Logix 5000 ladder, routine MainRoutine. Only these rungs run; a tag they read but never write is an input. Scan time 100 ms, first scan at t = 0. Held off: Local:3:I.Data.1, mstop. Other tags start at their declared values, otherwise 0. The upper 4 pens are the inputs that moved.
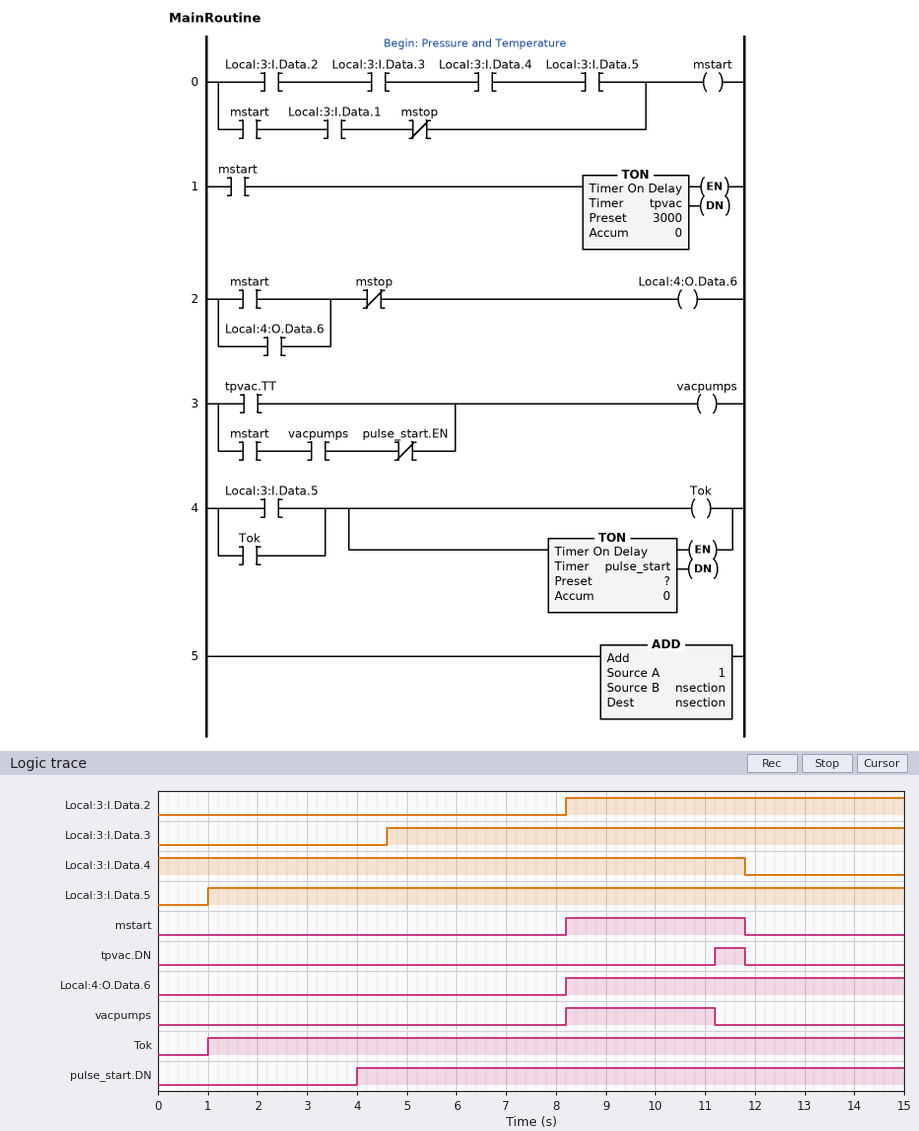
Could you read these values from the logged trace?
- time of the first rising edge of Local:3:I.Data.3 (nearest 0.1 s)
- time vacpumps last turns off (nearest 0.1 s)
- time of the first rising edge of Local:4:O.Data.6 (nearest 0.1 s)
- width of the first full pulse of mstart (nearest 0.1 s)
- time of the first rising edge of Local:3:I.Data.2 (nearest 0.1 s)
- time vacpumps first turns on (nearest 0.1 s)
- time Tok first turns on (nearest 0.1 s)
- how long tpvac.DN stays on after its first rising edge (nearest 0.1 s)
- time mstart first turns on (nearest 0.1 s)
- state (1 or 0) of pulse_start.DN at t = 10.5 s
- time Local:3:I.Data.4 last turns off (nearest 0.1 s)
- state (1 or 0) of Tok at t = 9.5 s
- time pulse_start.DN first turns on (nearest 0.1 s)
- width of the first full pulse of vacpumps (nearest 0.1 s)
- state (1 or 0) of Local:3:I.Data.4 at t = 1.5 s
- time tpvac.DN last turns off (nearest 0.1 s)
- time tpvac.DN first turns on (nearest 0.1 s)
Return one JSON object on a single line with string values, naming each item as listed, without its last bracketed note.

{"time of the first rising edge of Local:3:I.Data.3": "4.6 s", "time vacpumps last turns off": "11.2 s", "time of the first rising edge of Local:4:O.Data.6": "8.2 s", "width of the first full pulse of mstart": "3.6 s", "time of the first rising edge of Local:3:I.Data.2": "8.2 s", "time vacpumps first turns on": "8.2 s", "time Tok first turns on": "1.0 s", "how long tpvac.DN stays on after its first rising edge": "0.6 s", "time mstart first turns on": "8.2 s", "state (1 or 0) of pulse_start.DN at t = 10.5 s": "1", "time Local:3:I.Data.4 last turns off": "11.8 s", "state (1 or 0) of Tok at t = 9.5 s": "1", "time pulse_start.DN first turns on": "4.0 s", "width of the first full pulse of vacpumps": "3.0 s", "state (1 or 0) of Local:3:I.Data.4 at t = 1.5 s": "1", "time tpvac.DN last turns off": "11.8 s", "time tpvac.DN first turns on": "11.2 s"}
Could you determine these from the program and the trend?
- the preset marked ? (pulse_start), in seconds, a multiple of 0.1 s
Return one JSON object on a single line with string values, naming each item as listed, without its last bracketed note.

{"the preset marked ? (pulse_start), in seconds, a multiple of 0.1 s": "3.0 s"}
